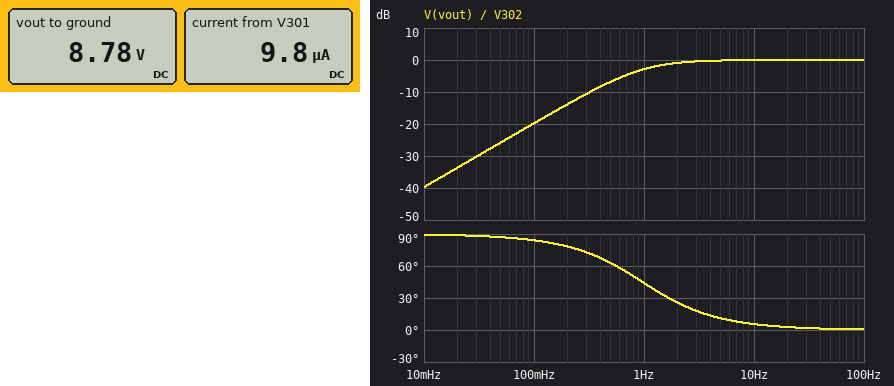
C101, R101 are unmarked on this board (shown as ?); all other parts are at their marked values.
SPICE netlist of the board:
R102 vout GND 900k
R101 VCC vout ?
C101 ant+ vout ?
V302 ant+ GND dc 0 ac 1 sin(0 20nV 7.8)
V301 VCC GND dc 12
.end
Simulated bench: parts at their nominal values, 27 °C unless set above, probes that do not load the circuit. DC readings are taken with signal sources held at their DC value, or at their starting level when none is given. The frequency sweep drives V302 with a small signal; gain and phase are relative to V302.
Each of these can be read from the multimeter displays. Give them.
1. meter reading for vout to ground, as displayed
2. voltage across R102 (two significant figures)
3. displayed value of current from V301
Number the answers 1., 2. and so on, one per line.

1. 8.78 V
2. 8.8 V
3. 9.8 µA
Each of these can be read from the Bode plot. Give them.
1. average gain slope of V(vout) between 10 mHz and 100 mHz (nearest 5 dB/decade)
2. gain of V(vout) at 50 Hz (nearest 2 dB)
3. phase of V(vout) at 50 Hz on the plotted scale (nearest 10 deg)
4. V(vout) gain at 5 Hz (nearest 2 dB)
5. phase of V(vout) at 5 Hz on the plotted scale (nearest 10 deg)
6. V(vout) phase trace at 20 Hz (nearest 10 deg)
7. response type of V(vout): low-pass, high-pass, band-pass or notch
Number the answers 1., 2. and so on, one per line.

1. 20 dB/decade
2. 0 dB
3. 0 deg
4. 0 dB
5. 10 deg
6. 0 deg
7. high-pass
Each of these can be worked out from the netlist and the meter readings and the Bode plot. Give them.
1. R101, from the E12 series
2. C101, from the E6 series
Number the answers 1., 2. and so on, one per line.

1. 330 kΩ
2. 680 nF
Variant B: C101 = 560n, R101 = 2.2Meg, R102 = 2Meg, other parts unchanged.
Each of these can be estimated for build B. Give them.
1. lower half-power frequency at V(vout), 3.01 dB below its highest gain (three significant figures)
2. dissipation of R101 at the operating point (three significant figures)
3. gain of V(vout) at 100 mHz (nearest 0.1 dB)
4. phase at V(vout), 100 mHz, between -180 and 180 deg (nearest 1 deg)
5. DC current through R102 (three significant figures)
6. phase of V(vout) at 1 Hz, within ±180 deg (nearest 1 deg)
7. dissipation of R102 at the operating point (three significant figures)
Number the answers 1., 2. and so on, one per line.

1. 271 mHz
2. 18.0 µW
3. -9.2 dB
4. 70 deg
5. 2.86 µA
6. 15 deg
7. 16.3 µW
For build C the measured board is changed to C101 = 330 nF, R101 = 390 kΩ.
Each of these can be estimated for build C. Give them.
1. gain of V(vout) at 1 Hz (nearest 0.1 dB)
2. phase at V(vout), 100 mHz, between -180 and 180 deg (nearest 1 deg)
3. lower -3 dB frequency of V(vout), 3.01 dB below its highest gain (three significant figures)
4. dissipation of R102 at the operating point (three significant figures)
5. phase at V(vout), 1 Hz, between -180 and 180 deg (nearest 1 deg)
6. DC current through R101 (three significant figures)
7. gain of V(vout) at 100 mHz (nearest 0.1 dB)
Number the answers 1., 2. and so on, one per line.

1. -6.2 dB
2. 87 deg
3. 1.77 Hz
4. 77.9 µW
5. 61 deg
6. 9.30 µA
7. -25.0 dB
